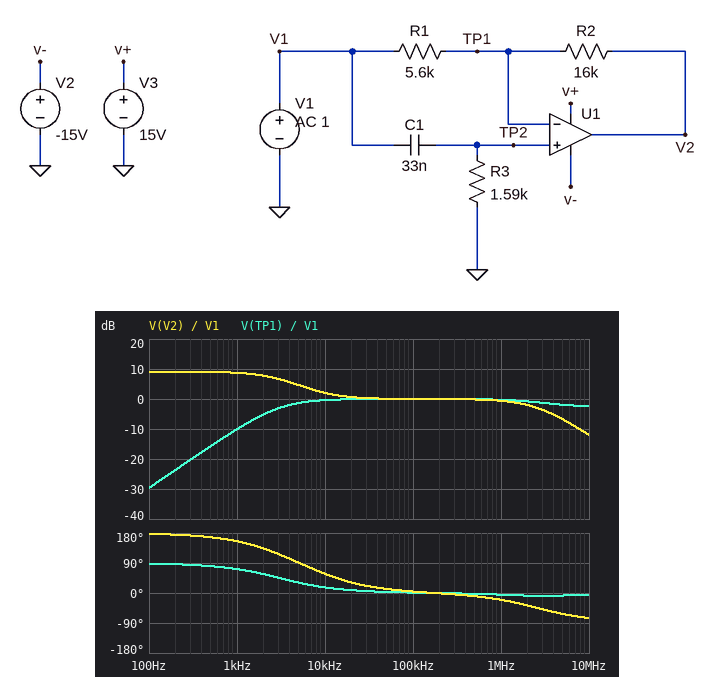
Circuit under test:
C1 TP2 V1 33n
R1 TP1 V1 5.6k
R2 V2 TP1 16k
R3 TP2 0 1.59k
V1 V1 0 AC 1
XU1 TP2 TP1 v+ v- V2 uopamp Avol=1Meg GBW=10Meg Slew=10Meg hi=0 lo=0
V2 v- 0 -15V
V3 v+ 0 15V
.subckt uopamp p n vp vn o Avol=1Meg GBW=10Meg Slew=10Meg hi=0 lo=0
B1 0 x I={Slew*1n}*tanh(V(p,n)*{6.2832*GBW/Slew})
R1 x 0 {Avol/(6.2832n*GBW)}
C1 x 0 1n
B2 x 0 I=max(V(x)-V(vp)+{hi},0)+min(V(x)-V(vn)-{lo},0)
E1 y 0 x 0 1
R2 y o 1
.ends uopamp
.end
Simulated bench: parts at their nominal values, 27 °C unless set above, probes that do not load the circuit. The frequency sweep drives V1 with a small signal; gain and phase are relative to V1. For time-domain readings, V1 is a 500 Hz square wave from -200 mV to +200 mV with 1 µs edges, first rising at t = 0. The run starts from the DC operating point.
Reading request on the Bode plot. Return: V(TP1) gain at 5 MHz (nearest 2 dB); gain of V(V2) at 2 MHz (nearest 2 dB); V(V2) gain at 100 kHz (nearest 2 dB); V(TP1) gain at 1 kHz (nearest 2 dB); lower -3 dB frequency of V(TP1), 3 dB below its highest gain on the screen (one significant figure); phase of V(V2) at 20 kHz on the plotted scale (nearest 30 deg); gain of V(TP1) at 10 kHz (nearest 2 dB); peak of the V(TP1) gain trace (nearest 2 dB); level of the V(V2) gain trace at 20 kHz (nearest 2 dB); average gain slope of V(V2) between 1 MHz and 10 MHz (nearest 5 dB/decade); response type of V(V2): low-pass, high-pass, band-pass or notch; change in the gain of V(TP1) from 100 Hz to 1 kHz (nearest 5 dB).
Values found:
-2 dB
-2 dB
0 dB
-10 dB
3 kHz
30 deg
0 dB
0 dB
0 dB
-10 dB/decade
low-pass
20 dB
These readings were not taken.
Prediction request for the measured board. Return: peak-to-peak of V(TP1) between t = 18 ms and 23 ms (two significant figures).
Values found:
790 mV
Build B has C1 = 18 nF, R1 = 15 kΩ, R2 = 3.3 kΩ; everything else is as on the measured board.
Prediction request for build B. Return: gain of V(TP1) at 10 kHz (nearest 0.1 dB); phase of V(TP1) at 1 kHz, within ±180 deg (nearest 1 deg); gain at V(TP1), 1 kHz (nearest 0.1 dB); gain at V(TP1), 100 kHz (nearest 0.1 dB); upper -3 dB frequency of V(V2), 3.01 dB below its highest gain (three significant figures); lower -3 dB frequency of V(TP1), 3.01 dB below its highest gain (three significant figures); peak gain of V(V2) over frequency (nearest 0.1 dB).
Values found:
-1.2 dB
80 deg
-15.0 dB
0 dB
8.21 MHz
5.55 kHz
0 dB
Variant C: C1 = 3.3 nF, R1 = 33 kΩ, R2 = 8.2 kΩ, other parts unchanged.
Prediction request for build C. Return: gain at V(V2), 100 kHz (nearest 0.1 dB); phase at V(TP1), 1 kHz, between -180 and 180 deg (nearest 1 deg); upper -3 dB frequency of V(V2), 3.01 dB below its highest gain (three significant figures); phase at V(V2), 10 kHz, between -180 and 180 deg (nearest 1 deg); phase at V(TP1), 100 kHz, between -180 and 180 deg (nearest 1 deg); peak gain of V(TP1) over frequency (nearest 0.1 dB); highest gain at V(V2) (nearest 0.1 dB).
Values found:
-0.4 dB
88 deg
8.07 MHz
109 deg
16 deg
0 dB
0 dB
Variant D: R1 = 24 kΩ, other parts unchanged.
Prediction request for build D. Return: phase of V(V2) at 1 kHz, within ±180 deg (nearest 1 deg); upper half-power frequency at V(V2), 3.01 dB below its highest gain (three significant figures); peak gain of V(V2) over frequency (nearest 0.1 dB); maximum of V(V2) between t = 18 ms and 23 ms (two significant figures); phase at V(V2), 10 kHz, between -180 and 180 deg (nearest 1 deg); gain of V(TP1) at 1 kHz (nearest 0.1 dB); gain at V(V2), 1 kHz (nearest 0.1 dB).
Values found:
135 deg
6.00 MHz
0 dB
530 mV
28 deg
-10.1 dB
-3.0 dB
